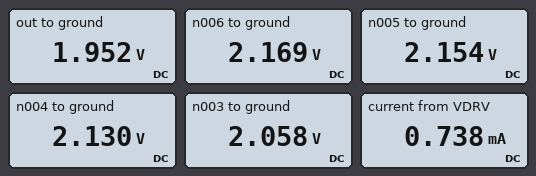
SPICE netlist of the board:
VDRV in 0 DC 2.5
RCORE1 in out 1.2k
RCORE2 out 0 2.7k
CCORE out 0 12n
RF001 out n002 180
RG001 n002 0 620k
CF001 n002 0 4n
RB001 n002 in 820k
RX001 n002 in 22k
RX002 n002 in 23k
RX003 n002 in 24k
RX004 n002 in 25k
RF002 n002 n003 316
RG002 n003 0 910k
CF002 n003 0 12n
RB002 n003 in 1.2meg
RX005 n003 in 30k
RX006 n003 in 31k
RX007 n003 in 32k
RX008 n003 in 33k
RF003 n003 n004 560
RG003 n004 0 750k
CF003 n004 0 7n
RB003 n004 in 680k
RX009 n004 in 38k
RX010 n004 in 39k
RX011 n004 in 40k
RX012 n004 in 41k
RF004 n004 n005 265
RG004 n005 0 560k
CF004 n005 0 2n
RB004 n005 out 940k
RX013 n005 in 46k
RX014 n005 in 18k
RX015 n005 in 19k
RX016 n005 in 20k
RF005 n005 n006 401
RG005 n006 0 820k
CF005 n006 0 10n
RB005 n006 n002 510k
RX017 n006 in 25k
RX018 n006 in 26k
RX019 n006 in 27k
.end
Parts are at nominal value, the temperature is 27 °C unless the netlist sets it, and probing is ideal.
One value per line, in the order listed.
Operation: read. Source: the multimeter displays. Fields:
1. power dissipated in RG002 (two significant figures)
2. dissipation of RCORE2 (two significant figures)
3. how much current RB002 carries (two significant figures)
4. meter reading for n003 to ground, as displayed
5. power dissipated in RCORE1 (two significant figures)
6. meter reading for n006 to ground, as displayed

4.7 µW
1.4 mW
370 nA
2.058 V
250 µW
2.169 V
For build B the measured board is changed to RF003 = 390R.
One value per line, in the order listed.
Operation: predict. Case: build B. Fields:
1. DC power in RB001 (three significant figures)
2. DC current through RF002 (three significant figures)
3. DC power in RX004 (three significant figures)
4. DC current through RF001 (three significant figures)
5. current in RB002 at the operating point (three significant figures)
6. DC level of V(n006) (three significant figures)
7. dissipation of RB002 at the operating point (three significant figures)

300 nW
188 µA
9.85 µW
270 µA
364 nA
2.16 V
159 nW
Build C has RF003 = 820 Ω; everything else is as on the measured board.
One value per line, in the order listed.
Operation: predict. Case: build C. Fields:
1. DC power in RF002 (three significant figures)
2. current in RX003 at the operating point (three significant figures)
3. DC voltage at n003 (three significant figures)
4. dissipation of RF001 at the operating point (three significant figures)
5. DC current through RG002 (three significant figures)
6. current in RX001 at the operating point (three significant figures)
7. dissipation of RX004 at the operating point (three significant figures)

9.84 µW
21.1 µA
2.05 V
12.2 µW
2.25 µA
23.0 µA
10.2 µW
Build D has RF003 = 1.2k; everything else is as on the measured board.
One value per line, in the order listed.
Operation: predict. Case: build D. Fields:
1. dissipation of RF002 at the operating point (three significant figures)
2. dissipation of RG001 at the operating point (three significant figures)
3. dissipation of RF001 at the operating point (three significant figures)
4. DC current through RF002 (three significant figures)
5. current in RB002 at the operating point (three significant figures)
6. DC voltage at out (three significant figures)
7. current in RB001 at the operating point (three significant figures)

8.94 µW
6.37 µW
11.6 µW
168 µA
383 nA
1.94 V
625 nA
